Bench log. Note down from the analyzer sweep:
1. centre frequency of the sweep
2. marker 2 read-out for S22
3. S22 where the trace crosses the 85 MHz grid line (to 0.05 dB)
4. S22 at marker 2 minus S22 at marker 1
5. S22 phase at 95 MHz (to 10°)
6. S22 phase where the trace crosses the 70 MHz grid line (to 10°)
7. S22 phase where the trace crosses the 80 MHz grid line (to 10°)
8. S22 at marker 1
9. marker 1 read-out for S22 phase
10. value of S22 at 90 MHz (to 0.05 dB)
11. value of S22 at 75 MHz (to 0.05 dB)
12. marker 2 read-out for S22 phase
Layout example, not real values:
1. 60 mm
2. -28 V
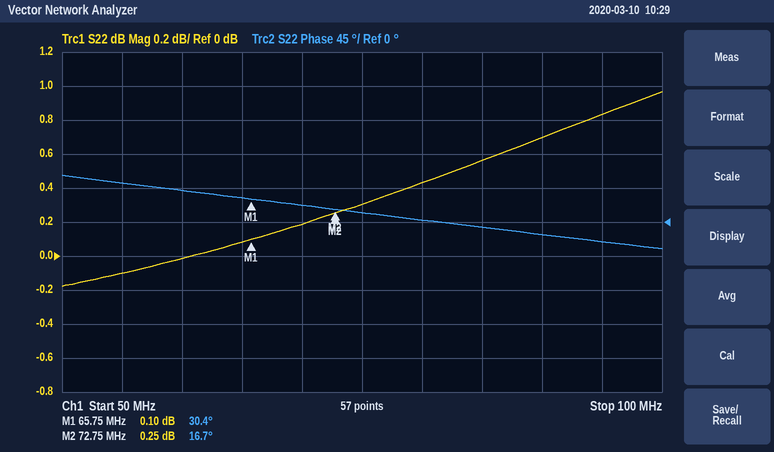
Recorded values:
1. 75 MHz
2. 0.25 dB
3. 0.55 dB
4. 0.15 dB
5. -30°
6. 20°
7. 0°
8. 0.10 dB
9. 30.4°
10. 0.70 dB
11. 0.30 dB
12. 16.7°
